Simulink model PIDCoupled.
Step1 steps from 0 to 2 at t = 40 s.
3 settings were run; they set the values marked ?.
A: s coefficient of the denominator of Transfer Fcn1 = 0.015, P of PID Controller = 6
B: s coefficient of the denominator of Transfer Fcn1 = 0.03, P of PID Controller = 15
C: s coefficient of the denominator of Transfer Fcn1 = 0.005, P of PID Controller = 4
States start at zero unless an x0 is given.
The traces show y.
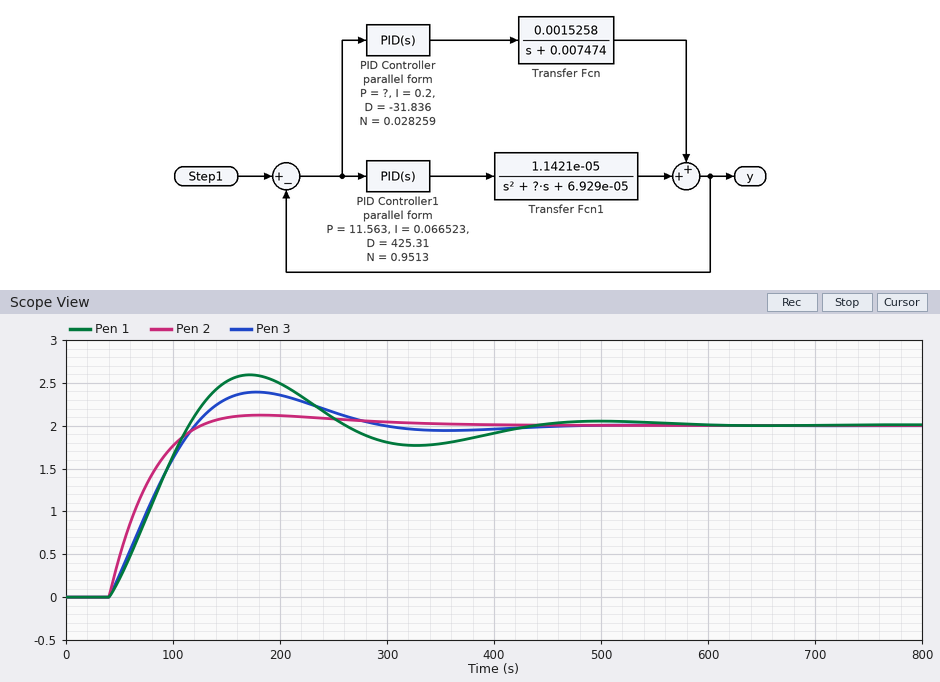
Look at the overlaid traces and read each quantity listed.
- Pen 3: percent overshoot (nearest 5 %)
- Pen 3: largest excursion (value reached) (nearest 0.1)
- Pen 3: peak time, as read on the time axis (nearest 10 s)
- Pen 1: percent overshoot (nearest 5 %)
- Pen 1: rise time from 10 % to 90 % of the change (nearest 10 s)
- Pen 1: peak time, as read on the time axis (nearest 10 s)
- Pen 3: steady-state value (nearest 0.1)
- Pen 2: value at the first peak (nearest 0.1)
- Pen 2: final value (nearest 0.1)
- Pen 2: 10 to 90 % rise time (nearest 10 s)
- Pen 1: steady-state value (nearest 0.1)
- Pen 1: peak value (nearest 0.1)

20 %
2.4
180 s
30 %
60 s
170 s
2.0
2.1
2.0
60 s
2.0
2.6
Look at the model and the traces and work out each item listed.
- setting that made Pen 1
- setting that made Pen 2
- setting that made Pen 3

C
B
A
